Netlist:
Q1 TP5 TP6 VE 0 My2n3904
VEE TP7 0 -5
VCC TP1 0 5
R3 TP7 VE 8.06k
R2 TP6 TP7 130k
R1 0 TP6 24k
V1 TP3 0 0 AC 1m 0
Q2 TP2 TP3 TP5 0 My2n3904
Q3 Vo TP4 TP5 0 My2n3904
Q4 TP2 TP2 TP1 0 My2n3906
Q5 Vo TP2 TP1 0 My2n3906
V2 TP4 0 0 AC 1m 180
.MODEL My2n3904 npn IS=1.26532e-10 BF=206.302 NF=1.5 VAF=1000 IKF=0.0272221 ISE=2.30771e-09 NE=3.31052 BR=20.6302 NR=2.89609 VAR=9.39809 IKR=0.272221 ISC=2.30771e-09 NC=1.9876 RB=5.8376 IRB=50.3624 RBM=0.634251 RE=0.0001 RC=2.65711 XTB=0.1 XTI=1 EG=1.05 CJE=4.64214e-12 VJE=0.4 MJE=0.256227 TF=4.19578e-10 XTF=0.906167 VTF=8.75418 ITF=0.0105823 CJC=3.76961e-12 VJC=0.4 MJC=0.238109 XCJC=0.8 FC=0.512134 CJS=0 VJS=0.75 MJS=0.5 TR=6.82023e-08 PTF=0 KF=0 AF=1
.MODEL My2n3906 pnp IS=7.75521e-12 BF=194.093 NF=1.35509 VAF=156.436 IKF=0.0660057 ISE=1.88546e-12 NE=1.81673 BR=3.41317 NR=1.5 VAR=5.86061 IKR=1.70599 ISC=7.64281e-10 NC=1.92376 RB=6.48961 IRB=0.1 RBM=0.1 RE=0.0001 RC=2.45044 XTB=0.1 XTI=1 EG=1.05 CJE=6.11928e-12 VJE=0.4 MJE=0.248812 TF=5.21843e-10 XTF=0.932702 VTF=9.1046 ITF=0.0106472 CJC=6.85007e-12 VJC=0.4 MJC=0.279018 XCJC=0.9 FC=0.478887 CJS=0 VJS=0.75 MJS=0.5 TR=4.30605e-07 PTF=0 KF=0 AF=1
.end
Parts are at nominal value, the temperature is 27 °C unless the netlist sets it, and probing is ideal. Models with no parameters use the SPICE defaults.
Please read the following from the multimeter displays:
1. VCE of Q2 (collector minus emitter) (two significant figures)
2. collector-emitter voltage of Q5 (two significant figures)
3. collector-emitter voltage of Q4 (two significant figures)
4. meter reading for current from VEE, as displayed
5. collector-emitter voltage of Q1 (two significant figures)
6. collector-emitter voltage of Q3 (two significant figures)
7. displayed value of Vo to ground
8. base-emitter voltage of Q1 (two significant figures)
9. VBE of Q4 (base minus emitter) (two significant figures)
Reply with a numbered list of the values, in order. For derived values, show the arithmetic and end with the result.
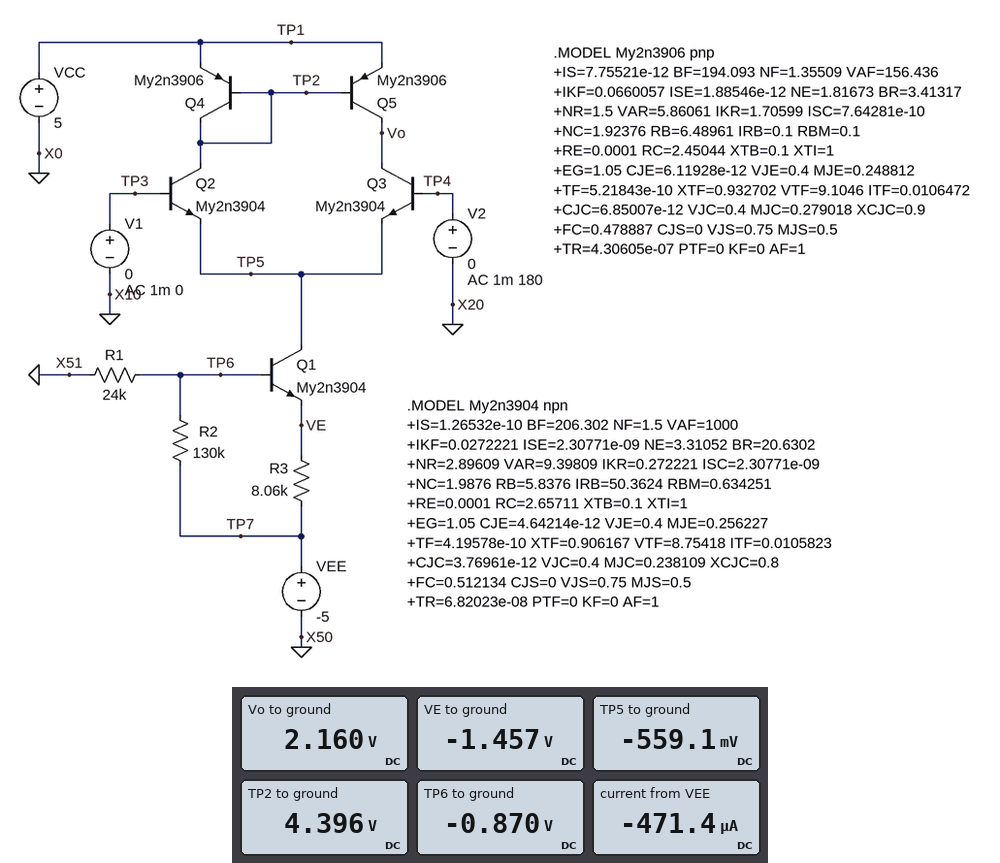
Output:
1. 4.396 V - (-559.1 mV) = 5.0 V
2. 2.16 V - 5 V = -2.8 V
3. 4.396 V - 5 V = -600 mV
4. -471.4 µA
5. -559.1 mV - (-1.457 V) = 900 mV
6. 2.16 V - (-559.1 mV) = 2.7 V
7. 2.160 V
8. -870 mV - (-1.457 V) = 590 mV
9. 4.396 V - 5 V = -600 mV
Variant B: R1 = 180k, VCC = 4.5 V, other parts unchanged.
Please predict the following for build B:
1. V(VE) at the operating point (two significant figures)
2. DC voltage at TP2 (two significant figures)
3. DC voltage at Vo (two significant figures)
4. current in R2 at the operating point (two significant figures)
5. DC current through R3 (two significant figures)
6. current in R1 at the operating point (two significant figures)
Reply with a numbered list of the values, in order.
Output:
1. -3.6 V
2. 3.9 V
3. 1.5 V
4. 15 µA
5. 170 µA
6. 17 µA
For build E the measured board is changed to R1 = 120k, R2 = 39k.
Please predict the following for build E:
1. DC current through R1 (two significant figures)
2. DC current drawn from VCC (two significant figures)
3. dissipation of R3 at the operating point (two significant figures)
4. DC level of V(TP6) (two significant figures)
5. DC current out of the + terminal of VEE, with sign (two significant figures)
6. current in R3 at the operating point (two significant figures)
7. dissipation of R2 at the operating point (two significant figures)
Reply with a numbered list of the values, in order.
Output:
1. 32 µA
2. 79 µA
3. 55 µW
4. -3.8 V
5. -110 µA
6. 82 µA
7. 36 µW
